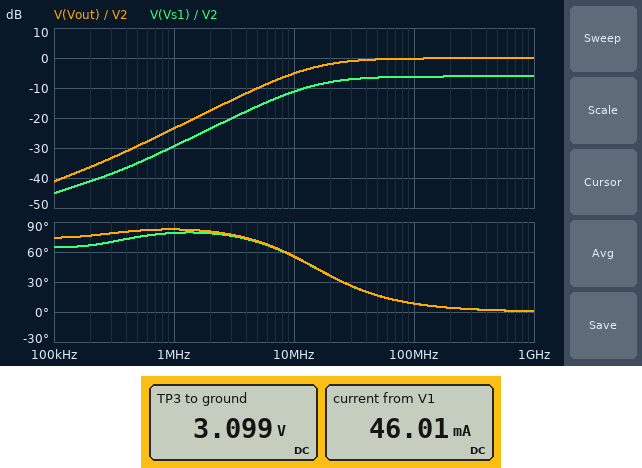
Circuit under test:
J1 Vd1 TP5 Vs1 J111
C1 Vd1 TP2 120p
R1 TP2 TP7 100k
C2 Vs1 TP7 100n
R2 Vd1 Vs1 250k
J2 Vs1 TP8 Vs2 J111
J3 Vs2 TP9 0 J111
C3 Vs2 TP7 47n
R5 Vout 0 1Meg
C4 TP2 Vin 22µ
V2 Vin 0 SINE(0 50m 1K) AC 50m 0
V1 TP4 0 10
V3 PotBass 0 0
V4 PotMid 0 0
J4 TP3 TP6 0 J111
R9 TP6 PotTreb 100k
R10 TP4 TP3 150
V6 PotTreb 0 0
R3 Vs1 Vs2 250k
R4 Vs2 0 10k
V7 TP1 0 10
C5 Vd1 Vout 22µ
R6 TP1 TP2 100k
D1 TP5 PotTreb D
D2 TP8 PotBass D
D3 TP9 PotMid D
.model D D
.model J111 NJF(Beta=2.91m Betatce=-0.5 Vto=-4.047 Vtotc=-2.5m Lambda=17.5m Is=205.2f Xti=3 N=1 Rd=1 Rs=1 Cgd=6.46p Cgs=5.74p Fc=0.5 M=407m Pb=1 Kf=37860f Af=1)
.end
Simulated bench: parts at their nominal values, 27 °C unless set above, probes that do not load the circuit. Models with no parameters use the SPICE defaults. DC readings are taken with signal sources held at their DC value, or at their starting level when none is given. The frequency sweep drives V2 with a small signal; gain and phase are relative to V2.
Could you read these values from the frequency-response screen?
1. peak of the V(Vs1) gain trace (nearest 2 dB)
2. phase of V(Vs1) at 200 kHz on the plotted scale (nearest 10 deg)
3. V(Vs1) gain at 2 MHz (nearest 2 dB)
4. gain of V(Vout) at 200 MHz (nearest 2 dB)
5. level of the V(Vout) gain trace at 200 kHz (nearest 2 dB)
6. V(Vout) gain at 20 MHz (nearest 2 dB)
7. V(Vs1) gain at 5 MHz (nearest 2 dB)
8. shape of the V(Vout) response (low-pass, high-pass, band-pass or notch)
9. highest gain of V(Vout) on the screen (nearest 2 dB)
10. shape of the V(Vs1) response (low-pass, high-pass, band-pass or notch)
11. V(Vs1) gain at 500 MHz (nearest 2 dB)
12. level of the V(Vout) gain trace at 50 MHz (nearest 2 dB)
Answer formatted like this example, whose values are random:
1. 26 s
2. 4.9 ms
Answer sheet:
1. -6 dB
2. 70 deg
3. -24 dB
4. 0 dB
5. -36 dB
6. -2 dB
7. -16 dB
8. high-pass
9. 0 dB
10. high-pass
11. -6 dB
12. 0 dB
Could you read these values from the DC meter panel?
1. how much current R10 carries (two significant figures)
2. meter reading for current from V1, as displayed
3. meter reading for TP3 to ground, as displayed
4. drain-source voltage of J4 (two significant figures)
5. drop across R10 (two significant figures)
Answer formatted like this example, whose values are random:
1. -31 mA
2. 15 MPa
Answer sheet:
1. 46 mA
2. 46.01 mA
3. 3.099 V
4. 3.1 V
5. 6.9 V
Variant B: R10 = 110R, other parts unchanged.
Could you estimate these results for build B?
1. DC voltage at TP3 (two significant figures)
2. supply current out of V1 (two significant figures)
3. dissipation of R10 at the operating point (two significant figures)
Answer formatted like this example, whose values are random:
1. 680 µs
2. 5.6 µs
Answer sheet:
1. 4.5 V
2. 50 mA
3. 280 mW
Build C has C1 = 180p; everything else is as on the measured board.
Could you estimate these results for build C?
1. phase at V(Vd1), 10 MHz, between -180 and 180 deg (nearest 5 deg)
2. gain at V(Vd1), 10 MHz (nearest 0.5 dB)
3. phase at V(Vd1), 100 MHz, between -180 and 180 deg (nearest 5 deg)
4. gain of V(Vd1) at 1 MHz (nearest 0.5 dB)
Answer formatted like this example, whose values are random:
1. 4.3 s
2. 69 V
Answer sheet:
1. 45 deg
2. -3.0 dB
3. 5 deg
4. -20.0 dB
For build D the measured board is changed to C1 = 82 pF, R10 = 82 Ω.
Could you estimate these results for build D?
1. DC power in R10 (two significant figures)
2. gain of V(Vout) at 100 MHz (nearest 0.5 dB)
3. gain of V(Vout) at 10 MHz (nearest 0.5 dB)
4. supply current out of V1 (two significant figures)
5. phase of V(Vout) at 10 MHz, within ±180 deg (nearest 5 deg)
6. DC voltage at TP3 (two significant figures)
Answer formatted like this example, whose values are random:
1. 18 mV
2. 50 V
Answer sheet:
1. 210 mW
2. -0.5 dB
3. -7.5 dB
4. 51 mA
5. 65 deg
6. 5.8 V
